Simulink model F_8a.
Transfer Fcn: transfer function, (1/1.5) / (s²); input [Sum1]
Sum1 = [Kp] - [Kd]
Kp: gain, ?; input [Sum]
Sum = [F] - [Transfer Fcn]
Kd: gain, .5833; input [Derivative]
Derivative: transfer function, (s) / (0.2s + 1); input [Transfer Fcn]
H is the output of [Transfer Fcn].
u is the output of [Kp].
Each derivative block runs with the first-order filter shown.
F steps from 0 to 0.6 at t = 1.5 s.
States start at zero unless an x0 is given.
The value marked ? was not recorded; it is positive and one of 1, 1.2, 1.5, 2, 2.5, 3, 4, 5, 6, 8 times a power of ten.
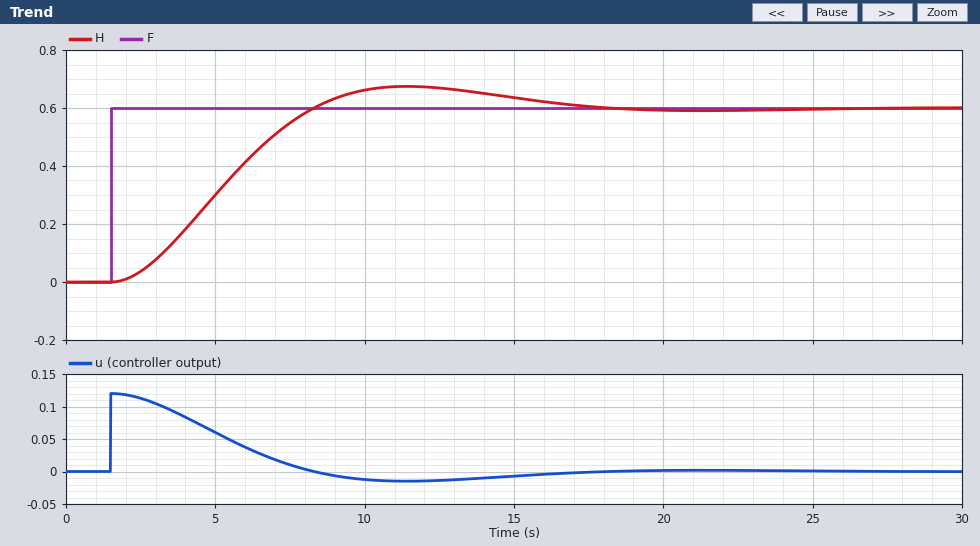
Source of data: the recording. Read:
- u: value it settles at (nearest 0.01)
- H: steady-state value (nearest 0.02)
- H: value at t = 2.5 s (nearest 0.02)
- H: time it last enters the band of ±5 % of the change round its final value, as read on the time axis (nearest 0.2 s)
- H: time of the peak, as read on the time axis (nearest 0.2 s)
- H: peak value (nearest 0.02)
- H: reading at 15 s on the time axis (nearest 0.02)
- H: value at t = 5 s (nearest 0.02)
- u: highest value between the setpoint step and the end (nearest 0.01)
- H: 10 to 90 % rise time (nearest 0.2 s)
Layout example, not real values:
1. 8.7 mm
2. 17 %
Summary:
1. 0.00
2. 0.60
3. 0.04
4. 15.4 s
5. 11.4 s
6. 0.68
7. 0.64
8. 0.30
9. 0.12
10. 4.6 s
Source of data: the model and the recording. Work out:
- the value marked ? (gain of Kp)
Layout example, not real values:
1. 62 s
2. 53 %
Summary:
1. 0.2
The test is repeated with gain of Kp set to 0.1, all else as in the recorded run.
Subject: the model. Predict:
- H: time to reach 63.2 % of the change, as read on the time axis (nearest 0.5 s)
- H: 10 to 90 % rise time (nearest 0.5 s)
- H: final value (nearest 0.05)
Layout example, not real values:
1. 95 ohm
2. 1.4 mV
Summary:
1. 8.5 s
2. 9.0 s
3. 0.60
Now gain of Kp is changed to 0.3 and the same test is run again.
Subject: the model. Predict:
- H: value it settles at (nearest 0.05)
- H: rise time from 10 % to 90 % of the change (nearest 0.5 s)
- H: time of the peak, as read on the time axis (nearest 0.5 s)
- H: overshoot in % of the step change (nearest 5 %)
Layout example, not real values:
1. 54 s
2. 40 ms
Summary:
1. 0.60
2. 3.5 s
3. 9.0 s
4. 20 %
